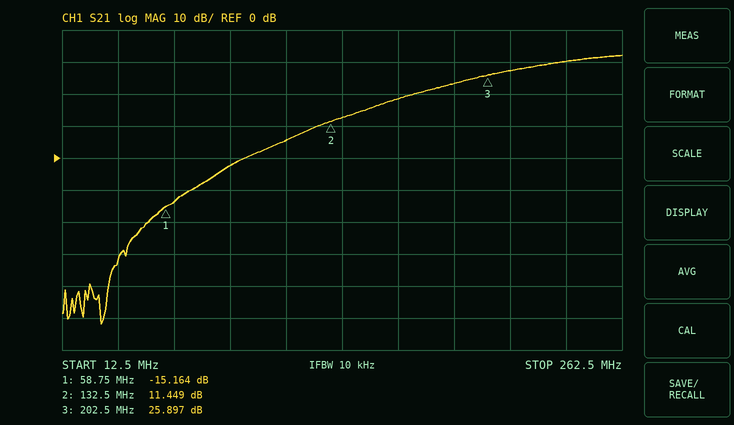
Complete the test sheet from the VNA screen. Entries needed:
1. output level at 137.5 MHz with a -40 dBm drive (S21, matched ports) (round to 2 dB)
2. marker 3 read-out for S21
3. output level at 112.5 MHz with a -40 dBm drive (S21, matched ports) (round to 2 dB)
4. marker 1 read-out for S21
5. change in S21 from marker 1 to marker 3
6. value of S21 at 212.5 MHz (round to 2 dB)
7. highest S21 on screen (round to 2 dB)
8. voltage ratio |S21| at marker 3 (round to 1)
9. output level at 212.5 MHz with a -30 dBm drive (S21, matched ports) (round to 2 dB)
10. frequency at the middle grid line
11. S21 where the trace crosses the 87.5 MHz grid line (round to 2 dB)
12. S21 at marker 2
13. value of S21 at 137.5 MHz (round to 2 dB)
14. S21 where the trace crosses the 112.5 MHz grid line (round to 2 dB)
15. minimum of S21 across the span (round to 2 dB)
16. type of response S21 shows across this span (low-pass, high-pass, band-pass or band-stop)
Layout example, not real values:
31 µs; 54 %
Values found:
-28 dBm; 25.897 dB; -34 dBm; -15.164 dB; 41.061 dB; 28 dB; 32 dB; 20; -2 dBm; 137.5 MHz; -2 dB; 11.449 dB; 12 dB; 6 dB; -52 dB; high-pass
